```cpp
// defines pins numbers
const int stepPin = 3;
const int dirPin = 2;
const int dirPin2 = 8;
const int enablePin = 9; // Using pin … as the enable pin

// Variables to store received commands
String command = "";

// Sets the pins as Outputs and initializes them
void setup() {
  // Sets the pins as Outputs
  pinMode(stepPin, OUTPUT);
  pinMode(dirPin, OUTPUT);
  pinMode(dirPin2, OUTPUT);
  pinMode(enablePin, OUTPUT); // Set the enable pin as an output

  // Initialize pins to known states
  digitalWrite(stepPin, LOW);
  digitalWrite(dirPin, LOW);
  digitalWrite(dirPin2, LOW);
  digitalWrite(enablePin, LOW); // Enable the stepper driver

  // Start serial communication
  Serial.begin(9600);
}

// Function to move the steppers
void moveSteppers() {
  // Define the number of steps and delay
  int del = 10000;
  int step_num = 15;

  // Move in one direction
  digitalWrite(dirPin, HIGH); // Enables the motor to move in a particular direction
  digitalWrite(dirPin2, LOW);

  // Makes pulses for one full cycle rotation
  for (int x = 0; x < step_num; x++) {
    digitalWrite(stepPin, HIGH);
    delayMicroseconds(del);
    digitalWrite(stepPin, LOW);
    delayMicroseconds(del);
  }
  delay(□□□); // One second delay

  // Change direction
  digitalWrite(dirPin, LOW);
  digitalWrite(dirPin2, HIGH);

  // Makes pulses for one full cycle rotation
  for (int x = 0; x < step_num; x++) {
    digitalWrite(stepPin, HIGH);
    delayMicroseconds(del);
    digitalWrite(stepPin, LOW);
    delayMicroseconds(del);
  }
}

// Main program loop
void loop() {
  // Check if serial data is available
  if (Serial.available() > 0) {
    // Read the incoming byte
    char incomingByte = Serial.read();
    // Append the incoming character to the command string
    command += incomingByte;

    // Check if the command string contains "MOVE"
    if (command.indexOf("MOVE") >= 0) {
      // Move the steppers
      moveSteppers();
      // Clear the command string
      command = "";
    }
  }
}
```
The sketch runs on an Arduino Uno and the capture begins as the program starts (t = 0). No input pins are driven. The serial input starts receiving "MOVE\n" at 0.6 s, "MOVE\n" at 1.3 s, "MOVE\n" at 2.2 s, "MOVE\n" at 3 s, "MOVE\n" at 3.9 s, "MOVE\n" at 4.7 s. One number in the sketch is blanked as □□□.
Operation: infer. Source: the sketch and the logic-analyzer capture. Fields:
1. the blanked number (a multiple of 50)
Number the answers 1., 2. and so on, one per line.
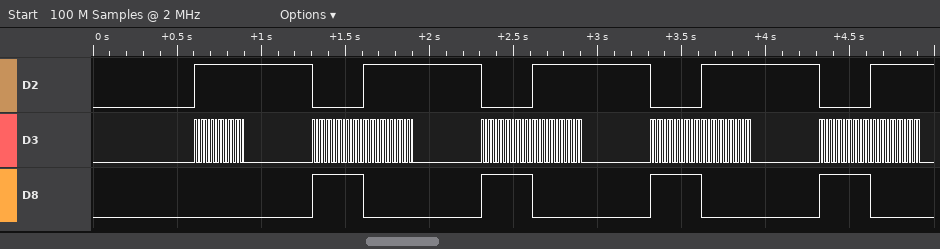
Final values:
1. 400
